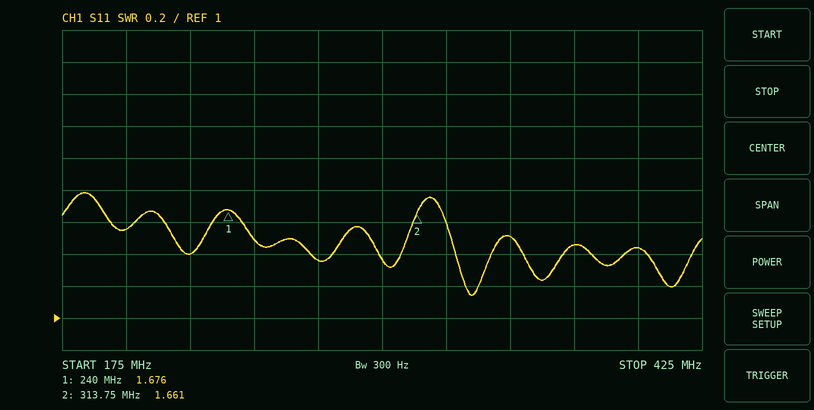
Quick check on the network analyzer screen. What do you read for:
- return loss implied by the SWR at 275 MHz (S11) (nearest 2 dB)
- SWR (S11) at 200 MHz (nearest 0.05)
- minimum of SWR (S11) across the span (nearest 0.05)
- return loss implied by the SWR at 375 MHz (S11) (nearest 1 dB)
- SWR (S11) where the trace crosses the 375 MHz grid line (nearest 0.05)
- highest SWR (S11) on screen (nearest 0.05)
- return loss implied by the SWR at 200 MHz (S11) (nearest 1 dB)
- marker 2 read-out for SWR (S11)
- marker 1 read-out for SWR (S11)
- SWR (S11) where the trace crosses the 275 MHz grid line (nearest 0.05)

16 dB
1.55
1.15
15 dB
1.45
1.80
13 dB
1.661
1.676
1.35
